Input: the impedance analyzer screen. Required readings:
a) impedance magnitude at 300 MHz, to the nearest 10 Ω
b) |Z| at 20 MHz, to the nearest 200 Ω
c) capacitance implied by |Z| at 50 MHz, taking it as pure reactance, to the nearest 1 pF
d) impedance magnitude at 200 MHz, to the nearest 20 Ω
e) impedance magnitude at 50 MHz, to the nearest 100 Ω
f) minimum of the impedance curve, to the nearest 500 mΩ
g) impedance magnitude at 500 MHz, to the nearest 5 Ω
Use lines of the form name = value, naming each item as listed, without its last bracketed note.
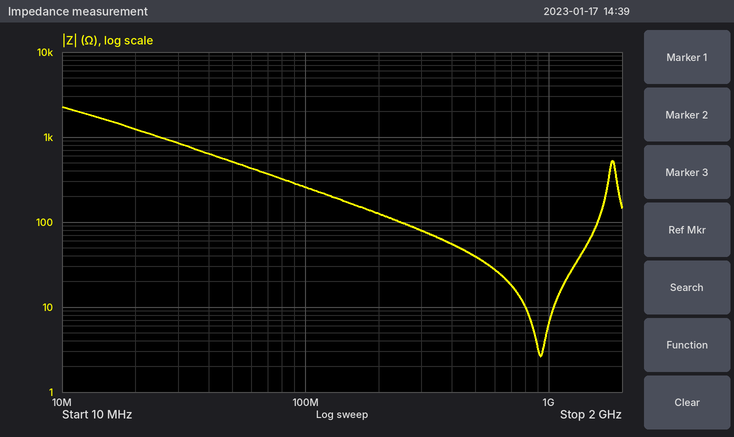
impedance magnitude at 300 MHz, to the nearest 10 Ω = 80 Ω
|Z| at 20 MHz, to the nearest 200 Ω = 1.2 kΩ
capacitance implied by |Z| at 50 MHz, taking it as pure reactance, to the nearest 1 pF = 6 pF
impedance magnitude at 200 MHz, to the nearest 20 Ω = 120 Ω
impedance magnitude at 50 MHz, to the nearest 100 Ω = 500 Ω
minimum of the impedance curve, to the nearest 500 mΩ = 2.5 Ω
impedance magnitude at 500 MHz, to the nearest 5 Ω = 40 Ω
